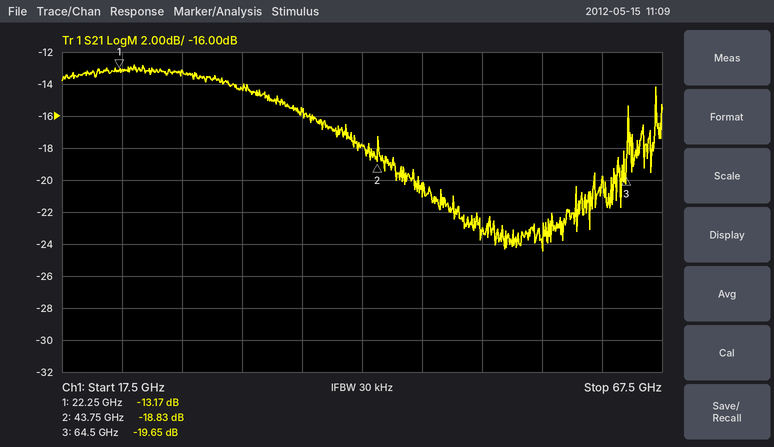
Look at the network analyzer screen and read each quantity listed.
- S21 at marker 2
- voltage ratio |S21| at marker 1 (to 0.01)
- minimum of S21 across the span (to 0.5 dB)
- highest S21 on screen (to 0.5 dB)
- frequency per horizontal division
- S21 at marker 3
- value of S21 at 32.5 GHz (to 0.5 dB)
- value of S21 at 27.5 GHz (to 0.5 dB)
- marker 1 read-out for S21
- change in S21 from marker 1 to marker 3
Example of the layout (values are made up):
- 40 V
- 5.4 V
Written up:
- -18.83 dB
- 0.22
- -24.5 dB
- -13.0 dB
- 5 GHz
- -19.65 dB
- -14.5 dB
- -13.0 dB
- -13.17 dB
- -6.48 dB
